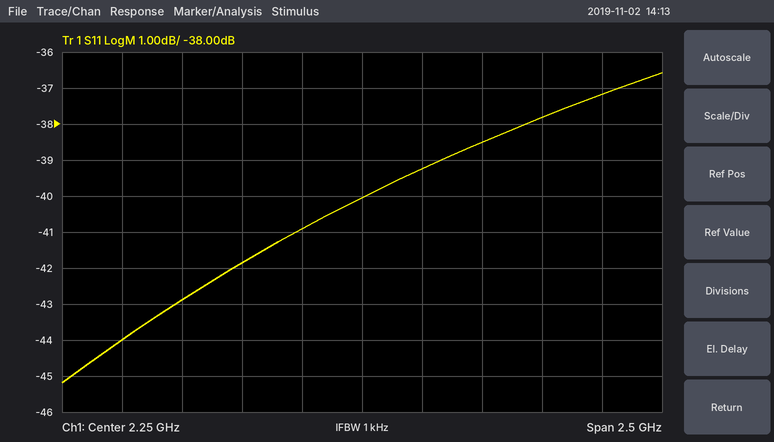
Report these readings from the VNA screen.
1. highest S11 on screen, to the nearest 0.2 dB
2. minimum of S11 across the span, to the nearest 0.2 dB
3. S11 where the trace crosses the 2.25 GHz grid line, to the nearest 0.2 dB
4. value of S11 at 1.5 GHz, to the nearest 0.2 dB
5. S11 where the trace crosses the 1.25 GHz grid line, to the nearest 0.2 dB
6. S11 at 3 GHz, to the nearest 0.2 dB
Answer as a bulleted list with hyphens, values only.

- -36.6 dB
- -45.2 dB
- -40.0 dB
- -42.8 dB
- -44.0 dB
- -37.8 dB
